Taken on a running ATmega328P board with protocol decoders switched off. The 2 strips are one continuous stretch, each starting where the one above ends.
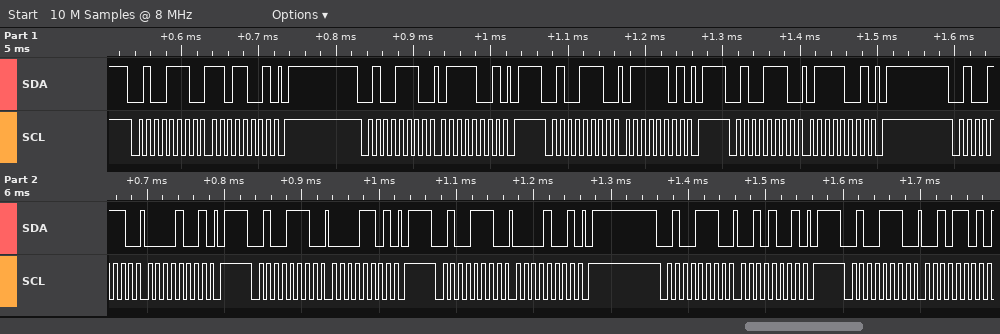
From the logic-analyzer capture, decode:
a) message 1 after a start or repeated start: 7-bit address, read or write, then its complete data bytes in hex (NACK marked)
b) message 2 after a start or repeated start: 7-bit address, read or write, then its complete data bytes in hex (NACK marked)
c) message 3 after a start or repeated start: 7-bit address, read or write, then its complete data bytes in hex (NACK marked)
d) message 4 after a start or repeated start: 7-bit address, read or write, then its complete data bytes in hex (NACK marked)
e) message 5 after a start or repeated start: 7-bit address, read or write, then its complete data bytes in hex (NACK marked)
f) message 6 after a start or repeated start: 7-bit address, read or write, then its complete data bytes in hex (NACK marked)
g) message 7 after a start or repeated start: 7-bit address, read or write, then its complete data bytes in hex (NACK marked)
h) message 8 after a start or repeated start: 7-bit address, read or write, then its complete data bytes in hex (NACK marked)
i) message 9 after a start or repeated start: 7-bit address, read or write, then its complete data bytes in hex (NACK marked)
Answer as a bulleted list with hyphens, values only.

- 0x27 write: D9
- 0x27 write: 79
- 0x27 write: 7D
- 0x27 write: 79
- 0x27 write: 09
- 0x27 write: 0D
- 0x27 write: 09
- 0x27 write: 29
- 0x27 write: 2D
